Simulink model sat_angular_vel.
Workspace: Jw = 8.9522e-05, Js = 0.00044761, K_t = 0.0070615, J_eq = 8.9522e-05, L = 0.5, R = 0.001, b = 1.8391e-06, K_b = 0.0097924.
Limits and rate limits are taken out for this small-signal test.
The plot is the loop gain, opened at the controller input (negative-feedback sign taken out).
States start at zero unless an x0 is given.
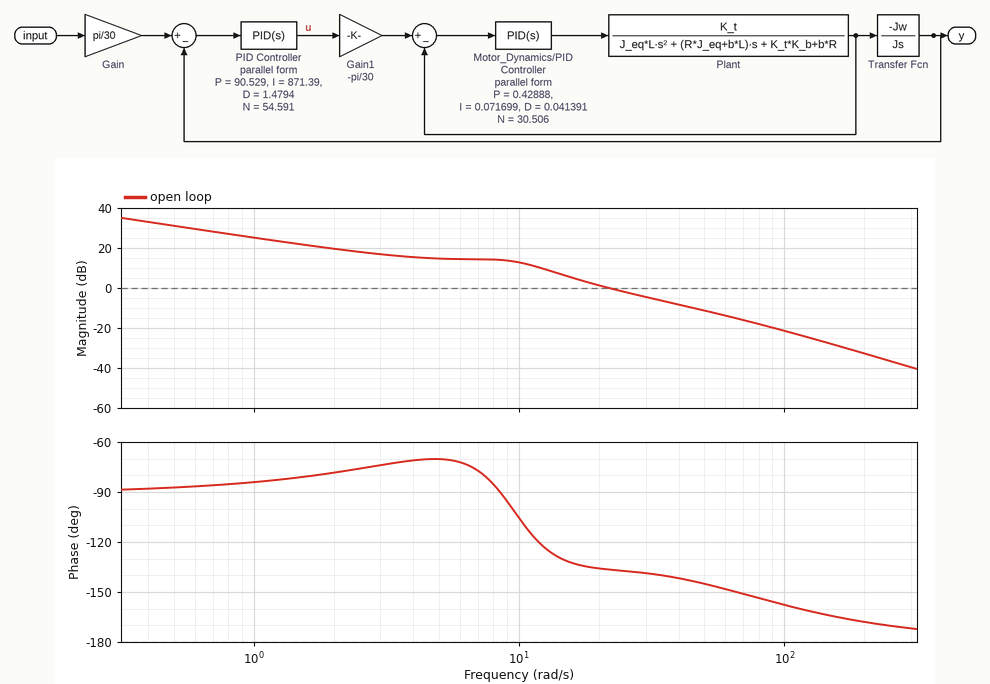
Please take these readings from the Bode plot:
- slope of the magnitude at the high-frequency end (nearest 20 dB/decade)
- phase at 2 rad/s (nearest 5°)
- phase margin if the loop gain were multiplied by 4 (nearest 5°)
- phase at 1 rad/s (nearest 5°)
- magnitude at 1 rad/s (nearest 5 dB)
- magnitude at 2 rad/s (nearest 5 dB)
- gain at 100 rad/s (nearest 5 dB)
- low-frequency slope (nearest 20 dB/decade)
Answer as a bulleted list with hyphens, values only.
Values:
- -40 dB/decade
- -80°
- 35°
- -85°
- 25 dB
- 20 dB
- -20 dB
- -20 dB/decade
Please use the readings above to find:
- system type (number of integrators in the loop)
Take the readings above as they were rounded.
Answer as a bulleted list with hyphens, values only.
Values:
- 1
